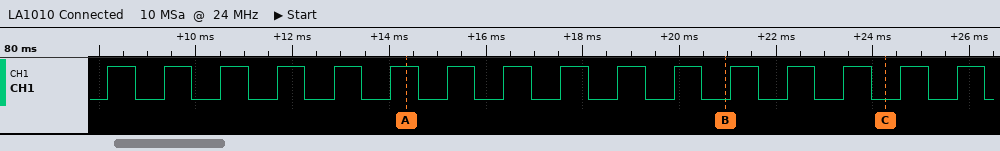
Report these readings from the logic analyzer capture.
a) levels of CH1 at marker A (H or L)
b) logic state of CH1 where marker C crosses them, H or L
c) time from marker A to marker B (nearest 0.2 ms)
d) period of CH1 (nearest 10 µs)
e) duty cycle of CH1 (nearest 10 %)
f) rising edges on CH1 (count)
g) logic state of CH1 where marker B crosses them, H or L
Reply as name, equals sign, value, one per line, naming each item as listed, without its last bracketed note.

levels of CH1 at marker A = CH1=H
logic state of CH1 where marker C crosses them, H or L = CH1=L
time from marker A to marker B = 6.6 ms
period of CH1 = 1170 µs
duty cycle of CH1 = 50 %
rising edges on CH1 = 16
logic state of CH1 where marker B crosses them, H or L = CH1=L
